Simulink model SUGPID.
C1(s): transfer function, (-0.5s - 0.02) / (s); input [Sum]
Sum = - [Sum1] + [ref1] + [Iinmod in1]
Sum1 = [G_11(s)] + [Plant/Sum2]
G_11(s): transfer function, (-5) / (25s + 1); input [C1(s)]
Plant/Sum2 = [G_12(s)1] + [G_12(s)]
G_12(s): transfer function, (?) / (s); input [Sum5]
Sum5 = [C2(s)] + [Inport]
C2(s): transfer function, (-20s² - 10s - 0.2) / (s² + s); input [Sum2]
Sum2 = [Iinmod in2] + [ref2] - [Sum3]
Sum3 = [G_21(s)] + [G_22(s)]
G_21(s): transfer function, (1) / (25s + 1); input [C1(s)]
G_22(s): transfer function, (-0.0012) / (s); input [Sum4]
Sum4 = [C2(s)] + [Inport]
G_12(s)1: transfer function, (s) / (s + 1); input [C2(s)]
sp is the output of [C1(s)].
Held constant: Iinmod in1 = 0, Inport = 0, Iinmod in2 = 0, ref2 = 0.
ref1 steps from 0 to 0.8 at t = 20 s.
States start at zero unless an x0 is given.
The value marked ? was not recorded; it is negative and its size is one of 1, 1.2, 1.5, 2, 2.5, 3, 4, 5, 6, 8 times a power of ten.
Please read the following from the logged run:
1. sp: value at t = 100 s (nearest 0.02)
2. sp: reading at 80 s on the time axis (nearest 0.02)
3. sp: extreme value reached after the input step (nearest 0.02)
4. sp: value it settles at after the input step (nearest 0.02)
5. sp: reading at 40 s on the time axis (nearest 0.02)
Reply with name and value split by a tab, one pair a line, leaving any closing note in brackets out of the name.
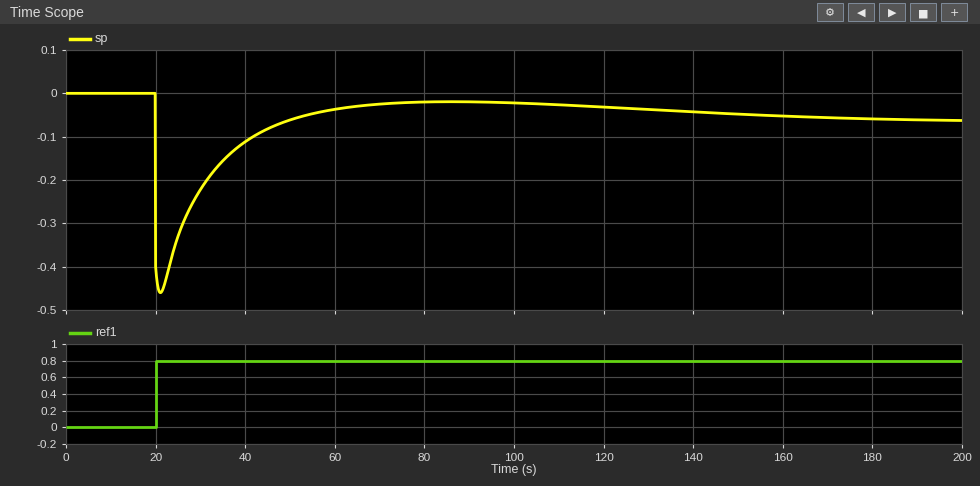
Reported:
sp: value at t = 100 s	-0.02
sp: reading at 80 s on the time axis	-0.02
sp: extreme value reached after the input step	-0.46
sp: value it settles at after the input step	-0.06
sp: reading at 40 s on the time axis	-0.12
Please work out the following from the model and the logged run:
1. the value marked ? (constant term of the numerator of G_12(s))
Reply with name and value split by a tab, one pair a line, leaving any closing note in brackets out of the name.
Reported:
the value marked ? (constant term of the numerator of G_12(s))	-0.01
